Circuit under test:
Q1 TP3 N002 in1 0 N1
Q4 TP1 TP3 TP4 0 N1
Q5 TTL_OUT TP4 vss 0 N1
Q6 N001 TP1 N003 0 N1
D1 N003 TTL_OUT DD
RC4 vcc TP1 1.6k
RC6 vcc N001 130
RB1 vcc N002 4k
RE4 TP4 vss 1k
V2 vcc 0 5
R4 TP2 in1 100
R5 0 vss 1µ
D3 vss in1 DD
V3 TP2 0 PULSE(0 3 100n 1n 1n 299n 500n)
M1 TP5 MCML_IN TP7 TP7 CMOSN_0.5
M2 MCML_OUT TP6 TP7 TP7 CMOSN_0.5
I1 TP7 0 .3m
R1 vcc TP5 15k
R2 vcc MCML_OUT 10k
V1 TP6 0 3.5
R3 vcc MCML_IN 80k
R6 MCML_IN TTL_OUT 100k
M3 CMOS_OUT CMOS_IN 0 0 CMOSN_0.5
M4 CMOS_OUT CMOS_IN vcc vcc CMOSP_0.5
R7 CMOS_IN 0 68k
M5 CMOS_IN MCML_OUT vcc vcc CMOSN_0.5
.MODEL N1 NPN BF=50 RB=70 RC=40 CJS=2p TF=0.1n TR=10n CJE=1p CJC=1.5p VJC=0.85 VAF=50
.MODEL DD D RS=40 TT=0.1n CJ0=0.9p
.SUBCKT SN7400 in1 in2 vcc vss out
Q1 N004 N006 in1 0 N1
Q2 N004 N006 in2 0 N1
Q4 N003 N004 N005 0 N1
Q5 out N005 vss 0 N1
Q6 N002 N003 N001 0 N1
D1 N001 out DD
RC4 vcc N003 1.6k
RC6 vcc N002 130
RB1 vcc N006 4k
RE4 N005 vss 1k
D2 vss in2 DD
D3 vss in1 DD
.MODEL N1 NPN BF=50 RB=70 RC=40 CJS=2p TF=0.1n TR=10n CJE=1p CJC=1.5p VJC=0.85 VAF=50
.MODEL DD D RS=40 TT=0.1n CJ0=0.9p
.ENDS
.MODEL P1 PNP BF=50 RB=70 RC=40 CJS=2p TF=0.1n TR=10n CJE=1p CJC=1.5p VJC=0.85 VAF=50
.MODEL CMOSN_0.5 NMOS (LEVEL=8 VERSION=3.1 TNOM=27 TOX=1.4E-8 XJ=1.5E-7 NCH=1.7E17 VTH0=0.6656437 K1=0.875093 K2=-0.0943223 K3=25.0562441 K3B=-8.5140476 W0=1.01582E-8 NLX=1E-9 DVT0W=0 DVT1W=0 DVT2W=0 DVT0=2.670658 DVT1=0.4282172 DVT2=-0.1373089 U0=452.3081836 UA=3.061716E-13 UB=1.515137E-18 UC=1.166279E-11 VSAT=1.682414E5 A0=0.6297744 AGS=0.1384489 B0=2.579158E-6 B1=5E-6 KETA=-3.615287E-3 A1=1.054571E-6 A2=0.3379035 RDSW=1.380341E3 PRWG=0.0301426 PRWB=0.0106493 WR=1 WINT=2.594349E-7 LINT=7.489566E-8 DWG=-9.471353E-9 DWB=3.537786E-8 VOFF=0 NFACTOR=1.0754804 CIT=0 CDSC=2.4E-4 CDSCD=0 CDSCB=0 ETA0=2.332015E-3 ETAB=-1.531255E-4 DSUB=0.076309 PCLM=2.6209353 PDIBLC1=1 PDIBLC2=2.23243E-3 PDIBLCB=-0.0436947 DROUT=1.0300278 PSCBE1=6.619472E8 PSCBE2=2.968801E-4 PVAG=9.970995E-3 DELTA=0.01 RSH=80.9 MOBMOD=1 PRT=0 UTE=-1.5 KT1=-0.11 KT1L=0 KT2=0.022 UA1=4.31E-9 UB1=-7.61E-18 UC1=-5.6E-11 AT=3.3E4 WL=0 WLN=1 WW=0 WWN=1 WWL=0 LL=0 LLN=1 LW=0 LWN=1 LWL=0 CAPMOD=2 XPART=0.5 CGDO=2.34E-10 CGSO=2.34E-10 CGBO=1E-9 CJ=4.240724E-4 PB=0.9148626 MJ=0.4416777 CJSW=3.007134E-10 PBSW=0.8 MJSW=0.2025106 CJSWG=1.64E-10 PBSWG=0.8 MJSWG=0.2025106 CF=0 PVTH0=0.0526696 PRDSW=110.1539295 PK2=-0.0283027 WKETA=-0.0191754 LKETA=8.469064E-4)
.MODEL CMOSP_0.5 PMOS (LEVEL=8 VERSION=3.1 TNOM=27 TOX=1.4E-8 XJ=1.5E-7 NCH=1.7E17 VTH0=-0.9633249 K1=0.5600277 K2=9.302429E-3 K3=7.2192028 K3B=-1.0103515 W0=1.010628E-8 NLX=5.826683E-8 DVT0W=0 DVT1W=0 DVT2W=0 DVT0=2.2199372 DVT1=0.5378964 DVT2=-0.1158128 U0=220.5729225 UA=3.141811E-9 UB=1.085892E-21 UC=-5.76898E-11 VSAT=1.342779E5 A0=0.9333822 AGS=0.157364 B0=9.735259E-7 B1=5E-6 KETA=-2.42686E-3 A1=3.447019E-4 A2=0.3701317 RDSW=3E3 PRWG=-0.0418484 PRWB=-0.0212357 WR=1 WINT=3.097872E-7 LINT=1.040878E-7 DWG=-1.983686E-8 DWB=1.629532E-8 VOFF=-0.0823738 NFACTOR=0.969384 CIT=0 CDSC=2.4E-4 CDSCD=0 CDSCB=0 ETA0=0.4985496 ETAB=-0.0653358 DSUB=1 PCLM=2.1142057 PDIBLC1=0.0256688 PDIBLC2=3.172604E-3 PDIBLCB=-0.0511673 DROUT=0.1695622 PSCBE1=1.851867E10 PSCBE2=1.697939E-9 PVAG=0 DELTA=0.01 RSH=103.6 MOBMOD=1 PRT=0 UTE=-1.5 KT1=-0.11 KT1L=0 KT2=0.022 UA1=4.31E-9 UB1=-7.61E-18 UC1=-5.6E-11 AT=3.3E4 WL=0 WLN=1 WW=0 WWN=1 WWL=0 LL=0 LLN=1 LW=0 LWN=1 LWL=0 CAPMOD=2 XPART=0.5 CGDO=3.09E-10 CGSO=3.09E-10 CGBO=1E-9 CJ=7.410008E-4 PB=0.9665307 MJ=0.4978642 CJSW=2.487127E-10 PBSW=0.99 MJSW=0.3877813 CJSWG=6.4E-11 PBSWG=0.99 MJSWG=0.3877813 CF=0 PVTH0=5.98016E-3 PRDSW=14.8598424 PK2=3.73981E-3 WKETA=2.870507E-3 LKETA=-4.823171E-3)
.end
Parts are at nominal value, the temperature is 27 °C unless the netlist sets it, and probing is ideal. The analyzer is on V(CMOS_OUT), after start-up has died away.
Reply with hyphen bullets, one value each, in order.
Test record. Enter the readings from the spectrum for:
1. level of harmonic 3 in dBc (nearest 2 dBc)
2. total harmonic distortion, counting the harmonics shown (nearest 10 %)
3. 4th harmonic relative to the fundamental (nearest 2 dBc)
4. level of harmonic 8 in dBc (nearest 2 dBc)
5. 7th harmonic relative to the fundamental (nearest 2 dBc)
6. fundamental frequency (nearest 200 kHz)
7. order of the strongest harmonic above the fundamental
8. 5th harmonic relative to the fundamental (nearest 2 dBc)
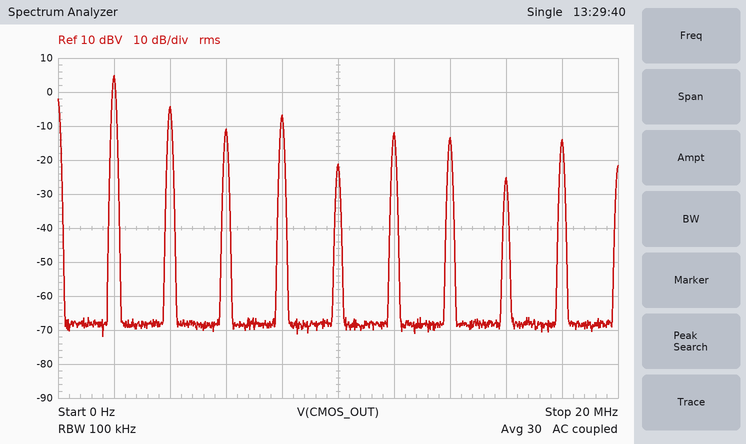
- -16 dBc
- 50 %
- -12 dBc
- -30 dBc
- -18 dBc
- 2.0 MHz
- 2
- -26 dBc
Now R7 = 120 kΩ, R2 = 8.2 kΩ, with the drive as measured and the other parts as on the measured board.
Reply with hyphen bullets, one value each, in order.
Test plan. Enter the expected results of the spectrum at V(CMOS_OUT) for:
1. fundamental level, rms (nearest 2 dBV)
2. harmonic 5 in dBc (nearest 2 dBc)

- -18 dBV
- -28 dBc
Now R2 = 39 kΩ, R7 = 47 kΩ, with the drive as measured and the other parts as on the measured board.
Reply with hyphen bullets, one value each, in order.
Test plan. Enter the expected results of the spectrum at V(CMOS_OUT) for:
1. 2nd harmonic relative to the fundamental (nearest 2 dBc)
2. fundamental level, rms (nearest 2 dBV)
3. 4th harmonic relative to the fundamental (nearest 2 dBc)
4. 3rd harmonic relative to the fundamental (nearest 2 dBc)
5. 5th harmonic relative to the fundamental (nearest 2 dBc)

- -2 dBc
- -66 dBV
- 0 dBc
- -8 dBc
- -8 dBc
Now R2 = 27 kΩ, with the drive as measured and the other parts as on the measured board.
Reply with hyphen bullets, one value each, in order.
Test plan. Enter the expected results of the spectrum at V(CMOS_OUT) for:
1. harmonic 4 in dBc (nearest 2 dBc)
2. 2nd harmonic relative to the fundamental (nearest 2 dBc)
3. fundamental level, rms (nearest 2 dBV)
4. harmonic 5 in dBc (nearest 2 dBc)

- -4 dBc
- -4 dBc
- -50 dBV
- -12 dBc
